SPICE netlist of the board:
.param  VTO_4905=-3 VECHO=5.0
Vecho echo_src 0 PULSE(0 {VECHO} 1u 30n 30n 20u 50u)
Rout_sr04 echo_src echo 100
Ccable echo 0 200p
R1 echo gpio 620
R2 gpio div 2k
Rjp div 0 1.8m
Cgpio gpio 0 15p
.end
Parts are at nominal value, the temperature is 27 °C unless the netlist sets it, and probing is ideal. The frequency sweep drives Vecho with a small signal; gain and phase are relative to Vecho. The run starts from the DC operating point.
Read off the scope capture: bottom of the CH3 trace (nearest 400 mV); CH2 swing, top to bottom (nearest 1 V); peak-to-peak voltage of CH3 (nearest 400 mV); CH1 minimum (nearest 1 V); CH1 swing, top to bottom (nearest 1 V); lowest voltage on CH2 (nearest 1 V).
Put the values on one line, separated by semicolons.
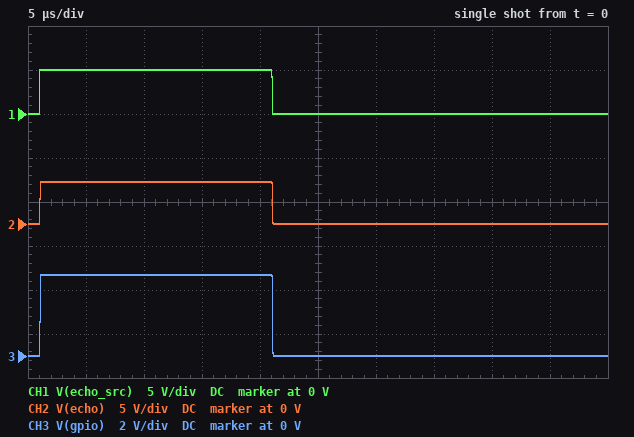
0 V; 5 V; 3.6 V; 0 V; 5 V; 0 V
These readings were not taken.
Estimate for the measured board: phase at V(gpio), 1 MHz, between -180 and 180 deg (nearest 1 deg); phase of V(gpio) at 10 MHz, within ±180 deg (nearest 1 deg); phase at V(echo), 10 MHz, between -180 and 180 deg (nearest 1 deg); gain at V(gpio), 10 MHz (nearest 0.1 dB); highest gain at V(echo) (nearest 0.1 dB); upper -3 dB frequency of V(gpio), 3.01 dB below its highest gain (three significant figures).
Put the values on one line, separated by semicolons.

-10 deg; -75 deg; -51 deg; -7.6 dB; -0.3 dB; 7.09 MHz
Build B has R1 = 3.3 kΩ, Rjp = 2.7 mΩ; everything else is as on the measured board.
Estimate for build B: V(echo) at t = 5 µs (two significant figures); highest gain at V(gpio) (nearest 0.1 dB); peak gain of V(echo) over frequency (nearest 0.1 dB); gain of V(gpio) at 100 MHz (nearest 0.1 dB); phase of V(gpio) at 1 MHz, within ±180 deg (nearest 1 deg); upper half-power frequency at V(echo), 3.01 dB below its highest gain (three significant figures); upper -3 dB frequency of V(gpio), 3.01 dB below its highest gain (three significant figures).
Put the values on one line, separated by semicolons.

4.9 V; -8.6 dB; -0.2 dB; -51.9 dB; -14 deg; 8.02 MHz; 5.31 MHz
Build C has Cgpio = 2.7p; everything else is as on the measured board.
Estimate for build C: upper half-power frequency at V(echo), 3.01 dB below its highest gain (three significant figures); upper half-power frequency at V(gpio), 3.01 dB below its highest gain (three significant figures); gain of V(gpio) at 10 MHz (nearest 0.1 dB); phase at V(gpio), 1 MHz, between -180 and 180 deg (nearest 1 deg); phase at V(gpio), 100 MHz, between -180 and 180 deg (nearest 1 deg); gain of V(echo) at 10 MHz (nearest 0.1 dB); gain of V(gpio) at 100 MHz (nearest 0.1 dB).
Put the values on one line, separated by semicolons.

8.19 MHz; 8.16 MHz; -6.7 dB; -7 deg; -124 deg; -4.3 dB; -26.6 dB
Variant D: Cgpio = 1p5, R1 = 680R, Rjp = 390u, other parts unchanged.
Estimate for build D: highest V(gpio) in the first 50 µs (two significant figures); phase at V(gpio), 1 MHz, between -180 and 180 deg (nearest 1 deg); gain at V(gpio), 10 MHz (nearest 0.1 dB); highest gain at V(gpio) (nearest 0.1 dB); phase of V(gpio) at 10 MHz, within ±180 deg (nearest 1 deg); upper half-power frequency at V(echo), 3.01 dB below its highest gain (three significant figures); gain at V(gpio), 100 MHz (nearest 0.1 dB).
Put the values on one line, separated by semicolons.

3.6 V; -7 deg; -6.8 dB; -2.9 dB; -53 deg; 8.22 MHz; -25.5 dB
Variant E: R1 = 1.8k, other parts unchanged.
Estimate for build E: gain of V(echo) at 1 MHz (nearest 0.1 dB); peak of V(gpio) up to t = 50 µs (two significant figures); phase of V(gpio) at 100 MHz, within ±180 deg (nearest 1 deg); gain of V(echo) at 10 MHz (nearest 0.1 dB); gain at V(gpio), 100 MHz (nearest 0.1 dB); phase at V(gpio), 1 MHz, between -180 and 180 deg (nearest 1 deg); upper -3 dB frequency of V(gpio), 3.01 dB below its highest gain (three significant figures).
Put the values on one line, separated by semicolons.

-0.3 dB; 2.6 V; -169 deg; -4.3 dB; -46.7 dB; -12 deg; 5.95 MHz
